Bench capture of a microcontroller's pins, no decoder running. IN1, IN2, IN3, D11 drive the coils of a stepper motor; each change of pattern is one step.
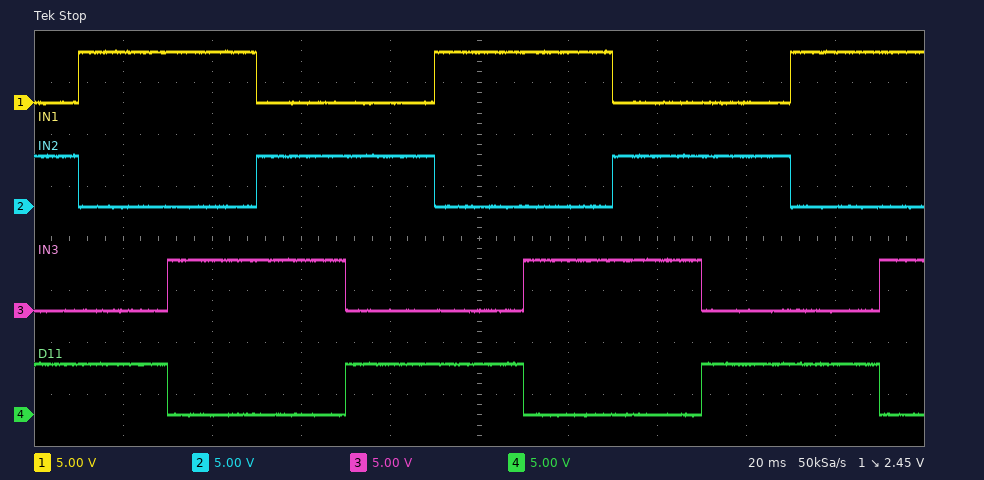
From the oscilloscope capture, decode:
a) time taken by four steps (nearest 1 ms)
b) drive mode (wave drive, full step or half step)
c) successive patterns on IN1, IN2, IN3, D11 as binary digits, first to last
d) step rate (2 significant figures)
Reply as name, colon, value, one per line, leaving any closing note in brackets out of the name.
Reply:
time taken by four steps: 80 ms
drive mode: full step
successive patterns on IN1, IN2, IN3, D11 as binary digits, first to last: 0101 1001 1010 0110 0101 1001 1010 0110 0101 1001 1010
step rate: 50 steps/s
